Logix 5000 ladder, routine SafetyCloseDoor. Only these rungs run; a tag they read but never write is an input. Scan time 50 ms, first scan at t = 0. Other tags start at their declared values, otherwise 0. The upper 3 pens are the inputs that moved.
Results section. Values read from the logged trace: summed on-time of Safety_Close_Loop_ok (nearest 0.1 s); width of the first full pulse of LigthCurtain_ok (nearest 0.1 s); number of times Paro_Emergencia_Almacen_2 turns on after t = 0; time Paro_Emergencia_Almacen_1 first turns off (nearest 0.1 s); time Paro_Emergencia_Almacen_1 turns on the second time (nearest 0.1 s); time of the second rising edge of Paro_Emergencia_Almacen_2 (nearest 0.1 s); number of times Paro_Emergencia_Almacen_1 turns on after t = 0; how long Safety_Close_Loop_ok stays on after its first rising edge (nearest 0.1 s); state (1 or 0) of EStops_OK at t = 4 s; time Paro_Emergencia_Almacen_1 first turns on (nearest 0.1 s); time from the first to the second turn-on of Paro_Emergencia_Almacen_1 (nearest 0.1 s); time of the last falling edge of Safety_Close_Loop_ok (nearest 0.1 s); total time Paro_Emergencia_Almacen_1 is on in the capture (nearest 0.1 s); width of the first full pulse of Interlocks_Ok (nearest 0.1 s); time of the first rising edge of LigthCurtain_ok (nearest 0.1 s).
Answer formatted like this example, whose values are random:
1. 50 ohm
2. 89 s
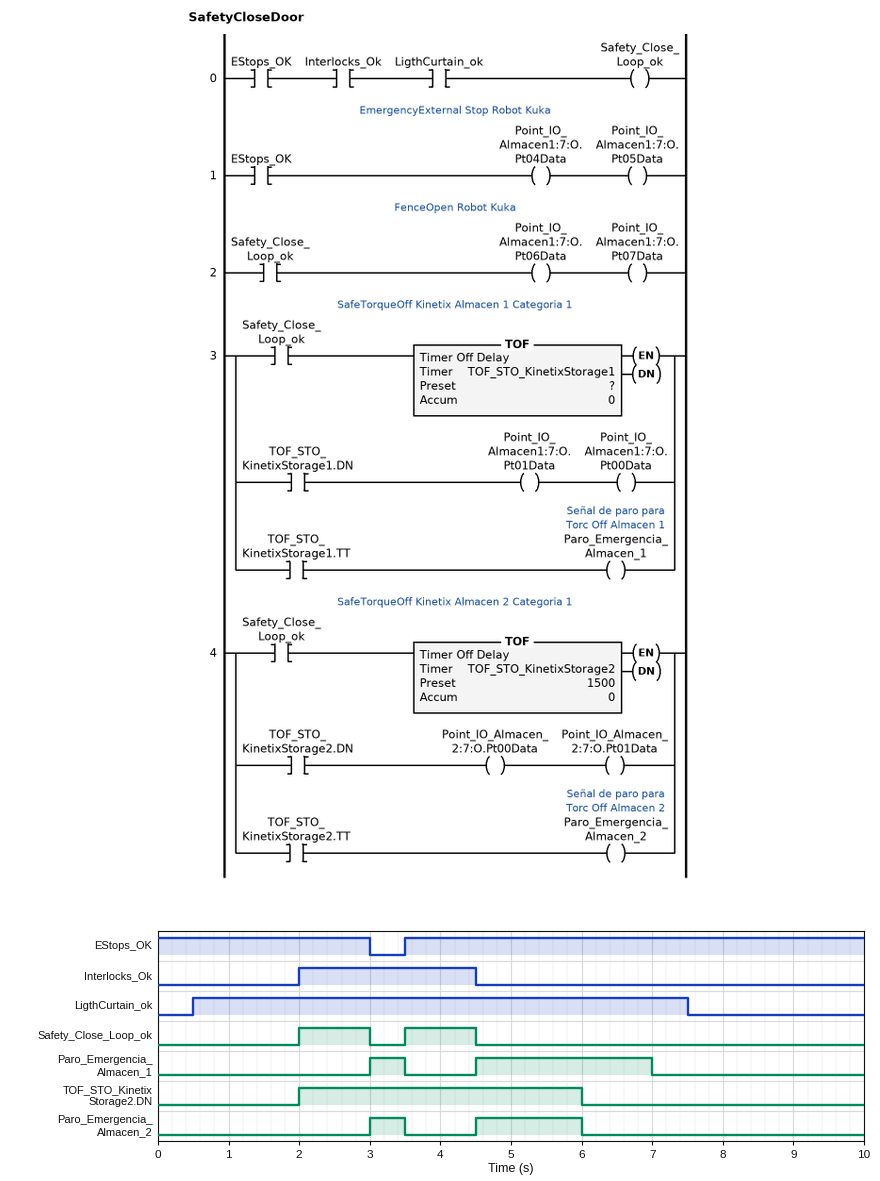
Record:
1. 2.0 s
2. 7.0 s
3. 2
4. 3.5 s
5. 4.5 s
6. 4.5 s
7. 2
8. 1.0 s
9. 1
10. 3.0 s
11. 1.5 s
12. 4.5 s
13. 3.0 s
14. 2.5 s
15. 0.5 s
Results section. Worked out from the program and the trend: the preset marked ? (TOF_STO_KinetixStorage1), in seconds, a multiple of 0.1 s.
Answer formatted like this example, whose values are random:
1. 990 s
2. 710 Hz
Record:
1. 2.5 s
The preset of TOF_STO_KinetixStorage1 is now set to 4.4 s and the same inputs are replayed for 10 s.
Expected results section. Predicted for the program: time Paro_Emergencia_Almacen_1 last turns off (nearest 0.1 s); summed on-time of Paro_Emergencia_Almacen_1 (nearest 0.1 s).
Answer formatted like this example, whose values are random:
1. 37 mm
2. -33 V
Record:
1. 8.9 s
2. 4.9 s
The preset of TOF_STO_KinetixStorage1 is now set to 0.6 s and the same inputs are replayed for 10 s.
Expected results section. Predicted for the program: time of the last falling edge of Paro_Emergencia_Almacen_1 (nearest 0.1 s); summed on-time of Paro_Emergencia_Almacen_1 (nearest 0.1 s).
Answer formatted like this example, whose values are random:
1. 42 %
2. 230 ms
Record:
1. 5.1 s
2. 1.1 s
